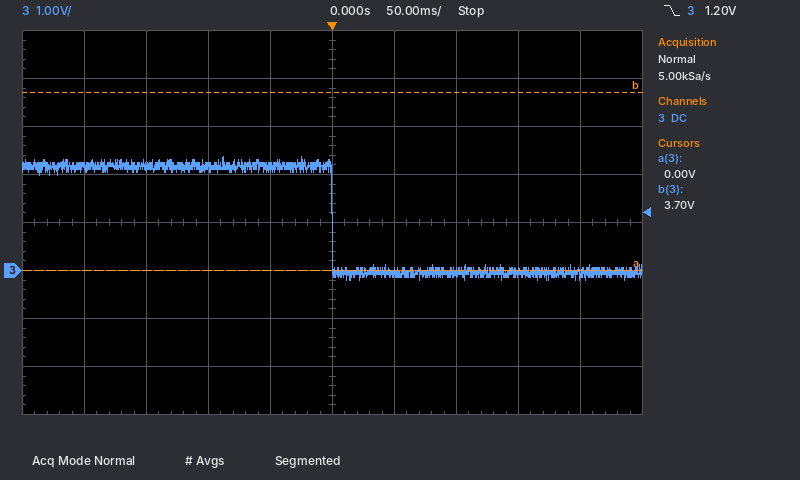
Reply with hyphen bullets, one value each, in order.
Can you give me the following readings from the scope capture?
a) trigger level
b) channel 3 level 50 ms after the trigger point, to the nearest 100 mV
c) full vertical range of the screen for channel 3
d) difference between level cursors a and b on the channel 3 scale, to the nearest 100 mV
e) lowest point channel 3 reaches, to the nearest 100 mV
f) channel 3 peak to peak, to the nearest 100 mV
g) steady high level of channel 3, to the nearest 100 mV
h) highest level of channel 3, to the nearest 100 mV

- 1.20 V
- 0.0 V
- 8 V
- 3.7 V
- -200 mV
- 2.6 V
- 2.2 V
- 2.4 V
